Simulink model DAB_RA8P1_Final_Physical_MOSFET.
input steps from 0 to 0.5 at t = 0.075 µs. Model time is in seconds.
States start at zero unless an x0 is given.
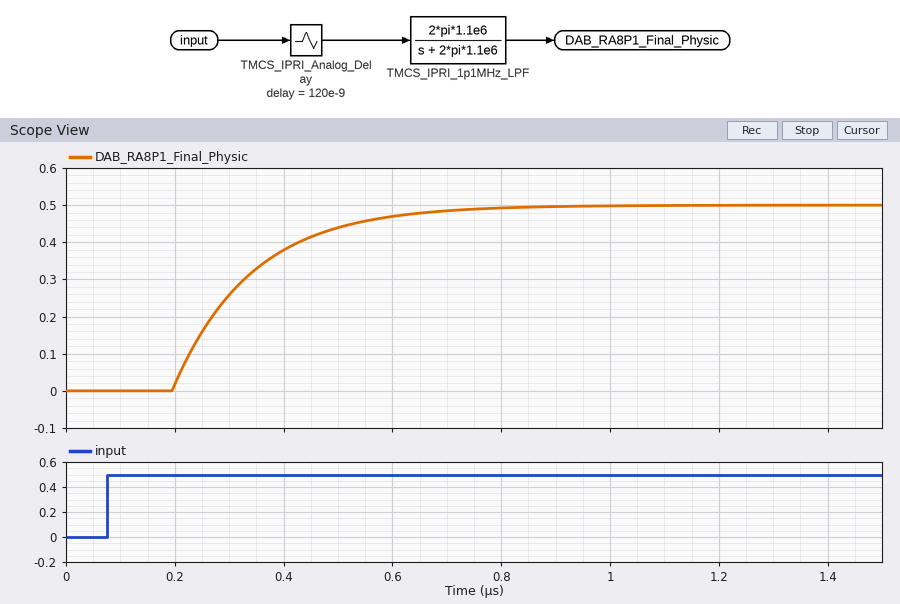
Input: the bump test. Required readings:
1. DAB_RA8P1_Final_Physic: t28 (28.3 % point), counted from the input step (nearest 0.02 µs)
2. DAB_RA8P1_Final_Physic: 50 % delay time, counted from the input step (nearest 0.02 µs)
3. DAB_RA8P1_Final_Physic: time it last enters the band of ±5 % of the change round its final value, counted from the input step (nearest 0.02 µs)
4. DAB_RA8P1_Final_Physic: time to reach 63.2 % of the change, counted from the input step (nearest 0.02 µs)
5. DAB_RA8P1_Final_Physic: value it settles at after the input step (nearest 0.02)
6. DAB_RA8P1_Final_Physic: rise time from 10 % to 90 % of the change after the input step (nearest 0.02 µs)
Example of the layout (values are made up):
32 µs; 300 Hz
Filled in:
0.16 µs; 0.22 µs; 0.56 µs; 0.26 µs; 0.50; 0.32 µs
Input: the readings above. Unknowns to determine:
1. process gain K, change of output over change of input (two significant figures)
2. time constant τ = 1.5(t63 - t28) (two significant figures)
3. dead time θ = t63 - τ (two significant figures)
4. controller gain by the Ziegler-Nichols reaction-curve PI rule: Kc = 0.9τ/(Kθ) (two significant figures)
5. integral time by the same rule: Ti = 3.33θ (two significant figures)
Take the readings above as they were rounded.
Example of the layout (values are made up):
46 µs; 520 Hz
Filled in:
1.0; 0.15 µs; 0.11 µs; 1.2; 0.37 µs
